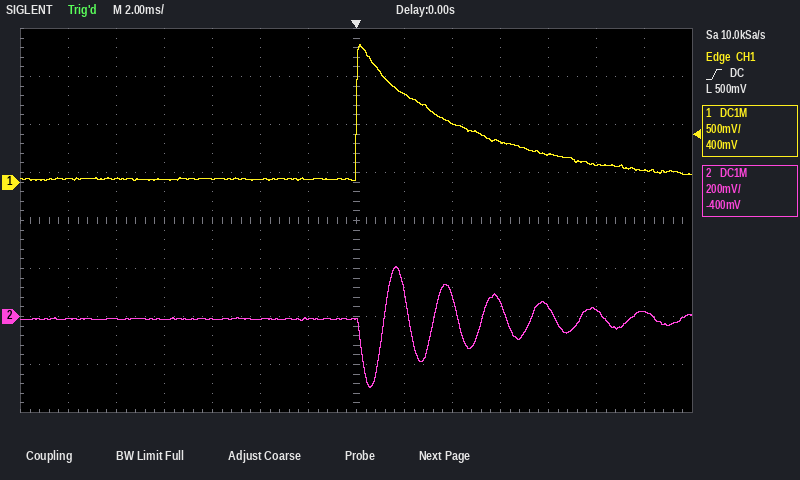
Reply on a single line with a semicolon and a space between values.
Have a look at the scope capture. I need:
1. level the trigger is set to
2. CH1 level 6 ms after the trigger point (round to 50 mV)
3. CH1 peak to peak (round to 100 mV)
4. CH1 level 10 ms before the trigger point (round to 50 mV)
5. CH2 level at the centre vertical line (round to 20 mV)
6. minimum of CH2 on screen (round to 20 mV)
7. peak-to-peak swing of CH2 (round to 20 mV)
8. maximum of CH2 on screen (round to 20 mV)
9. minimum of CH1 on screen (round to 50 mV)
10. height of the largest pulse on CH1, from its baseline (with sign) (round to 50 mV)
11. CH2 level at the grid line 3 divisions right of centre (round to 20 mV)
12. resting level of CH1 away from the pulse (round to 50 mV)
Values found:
500 mV; 400 mV; 1.40 V; 50 mV; -20 mV; -300 mV; 500 mV; 200 mV; 0 mV; +1.40 V; 60 mV; 50 mV
